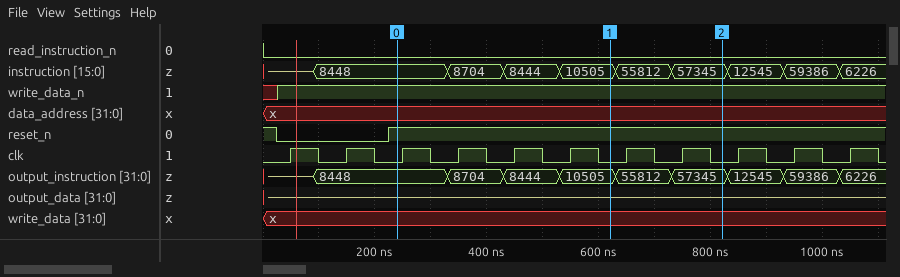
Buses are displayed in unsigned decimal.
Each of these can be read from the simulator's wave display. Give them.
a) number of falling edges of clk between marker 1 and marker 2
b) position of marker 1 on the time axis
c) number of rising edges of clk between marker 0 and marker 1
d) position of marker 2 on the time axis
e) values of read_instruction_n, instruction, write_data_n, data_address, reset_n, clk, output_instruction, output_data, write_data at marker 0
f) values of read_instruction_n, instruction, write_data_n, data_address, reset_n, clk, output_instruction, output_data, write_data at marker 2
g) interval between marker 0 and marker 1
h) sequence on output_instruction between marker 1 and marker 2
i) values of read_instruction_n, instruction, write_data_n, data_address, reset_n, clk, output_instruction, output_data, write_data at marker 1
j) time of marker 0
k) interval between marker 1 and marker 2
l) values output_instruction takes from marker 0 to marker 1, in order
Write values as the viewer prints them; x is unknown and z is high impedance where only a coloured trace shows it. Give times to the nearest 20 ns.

2
620 ns
4
820 ns
read_instruction_n=0, instruction=8448, write_data_n=1, data_address=x, reset_n=1, clk=0, output_instruction=8448, output_data=z, write_data=x
read_instruction_n=0, instruction=57345, write_data_n=1, data_address=x, reset_n=1, clk=0, output_instruction=57345, output_data=z, write_data=x
380 ns
10505, 55812, 57345
read_instruction_n=0, instruction=10505, write_data_n=1, data_address=x, reset_n=1, clk=0, output_instruction=10505, output_data=z, write_data=x
240 ns
200 ns
8448, 8704, 8444, 10505
